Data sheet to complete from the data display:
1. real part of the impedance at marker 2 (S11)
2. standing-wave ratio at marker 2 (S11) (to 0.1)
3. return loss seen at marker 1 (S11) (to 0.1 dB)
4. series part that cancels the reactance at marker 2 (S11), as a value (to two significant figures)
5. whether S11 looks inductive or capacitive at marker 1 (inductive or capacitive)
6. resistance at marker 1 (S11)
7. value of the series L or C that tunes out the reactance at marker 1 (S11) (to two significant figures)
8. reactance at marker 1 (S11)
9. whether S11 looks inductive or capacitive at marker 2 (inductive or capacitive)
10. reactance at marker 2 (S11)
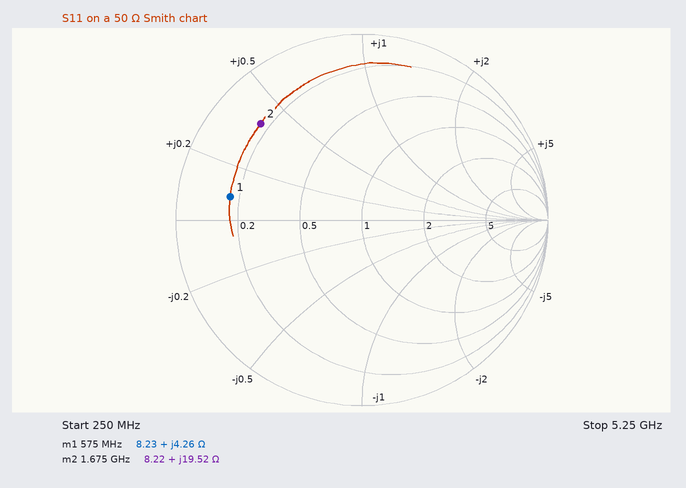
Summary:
8.22 Ω
7.0
2.9 dB
4.9 pF
inductive
8.23 Ω
65 pF
+4.26 Ω
inductive
+19.52 Ω
